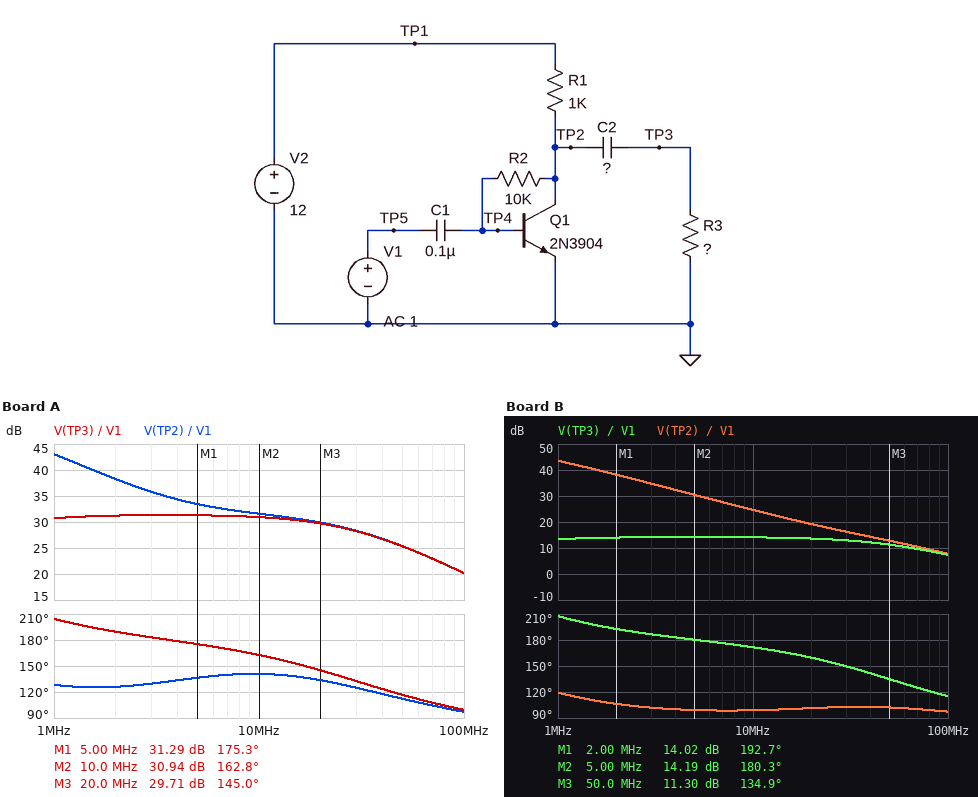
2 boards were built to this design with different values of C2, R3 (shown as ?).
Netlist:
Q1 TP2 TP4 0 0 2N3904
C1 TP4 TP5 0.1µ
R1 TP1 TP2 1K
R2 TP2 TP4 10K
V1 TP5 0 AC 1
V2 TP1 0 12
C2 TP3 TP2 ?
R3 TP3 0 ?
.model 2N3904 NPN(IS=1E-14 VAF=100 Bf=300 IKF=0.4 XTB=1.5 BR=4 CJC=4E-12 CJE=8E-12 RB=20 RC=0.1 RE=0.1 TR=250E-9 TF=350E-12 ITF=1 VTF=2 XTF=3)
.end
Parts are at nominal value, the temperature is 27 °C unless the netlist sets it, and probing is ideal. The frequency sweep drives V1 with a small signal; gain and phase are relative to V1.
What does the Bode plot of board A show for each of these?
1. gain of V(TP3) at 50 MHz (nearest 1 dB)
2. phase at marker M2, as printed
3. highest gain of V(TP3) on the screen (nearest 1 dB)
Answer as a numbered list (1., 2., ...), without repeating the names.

1. 25 dB
2. 162.8 deg
3. 31 dB
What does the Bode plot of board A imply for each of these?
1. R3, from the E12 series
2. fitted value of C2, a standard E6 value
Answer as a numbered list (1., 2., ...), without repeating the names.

1. 120 Ω
2. 330 pF
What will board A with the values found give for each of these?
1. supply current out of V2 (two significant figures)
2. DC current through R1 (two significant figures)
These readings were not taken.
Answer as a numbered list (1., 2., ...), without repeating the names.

1. 11 mA
2. 11 mA
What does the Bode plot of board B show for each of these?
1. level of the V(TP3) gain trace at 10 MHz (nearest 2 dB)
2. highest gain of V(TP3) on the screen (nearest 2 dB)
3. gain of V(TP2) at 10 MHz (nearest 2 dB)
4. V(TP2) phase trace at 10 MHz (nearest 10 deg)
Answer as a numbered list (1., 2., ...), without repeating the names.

1. 14 dB
2. 14 dB
3. 24 dB
4. 100 deg
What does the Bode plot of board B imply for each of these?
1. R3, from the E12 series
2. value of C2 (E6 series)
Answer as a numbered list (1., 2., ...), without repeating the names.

1. 15 Ω
2. 330 pF
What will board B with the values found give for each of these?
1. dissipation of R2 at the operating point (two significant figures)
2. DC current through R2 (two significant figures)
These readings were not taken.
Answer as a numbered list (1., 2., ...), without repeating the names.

1. 14 µW
2. 37 µA
